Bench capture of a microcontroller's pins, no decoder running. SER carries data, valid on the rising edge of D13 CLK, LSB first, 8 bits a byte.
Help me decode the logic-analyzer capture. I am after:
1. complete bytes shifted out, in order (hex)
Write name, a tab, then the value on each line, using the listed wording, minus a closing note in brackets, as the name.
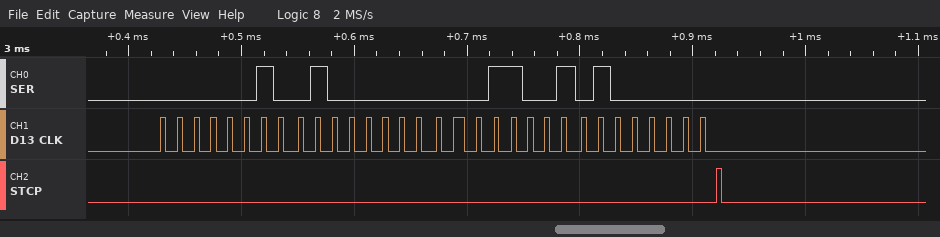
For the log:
complete bytes shifted out, in order	40 02 98 02
